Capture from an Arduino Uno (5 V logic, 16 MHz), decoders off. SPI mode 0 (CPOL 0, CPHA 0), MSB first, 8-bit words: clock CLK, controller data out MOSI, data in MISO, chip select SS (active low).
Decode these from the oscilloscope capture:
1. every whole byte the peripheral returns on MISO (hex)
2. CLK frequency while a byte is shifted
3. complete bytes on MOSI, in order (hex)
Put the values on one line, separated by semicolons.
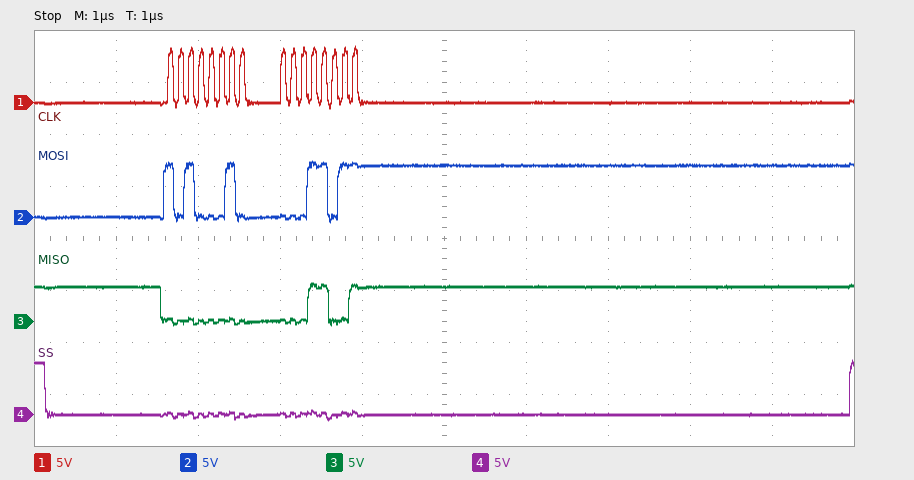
00 19; 8 MHz; A2 1B
